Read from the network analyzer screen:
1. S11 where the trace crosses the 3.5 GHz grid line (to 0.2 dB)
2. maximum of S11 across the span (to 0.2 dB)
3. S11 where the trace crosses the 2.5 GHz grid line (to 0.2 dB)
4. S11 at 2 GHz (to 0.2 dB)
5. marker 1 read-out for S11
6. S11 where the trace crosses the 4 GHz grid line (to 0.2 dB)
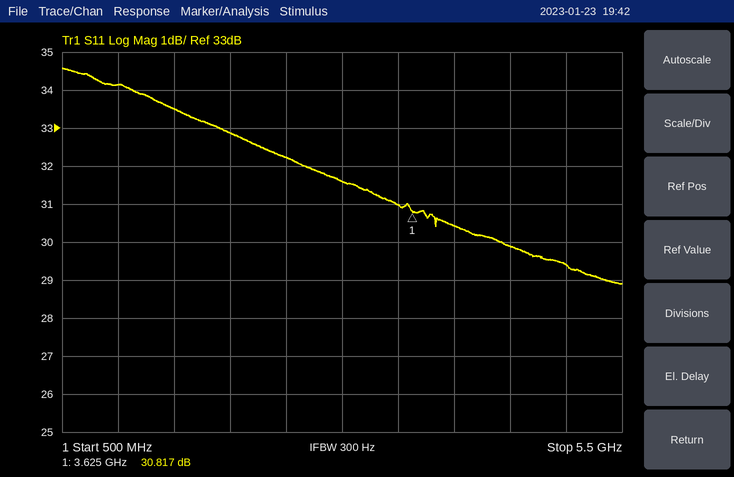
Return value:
31.0 dB
34.6 dB
32.2 dB
32.8 dB
30.817 dB
30.4 dB
